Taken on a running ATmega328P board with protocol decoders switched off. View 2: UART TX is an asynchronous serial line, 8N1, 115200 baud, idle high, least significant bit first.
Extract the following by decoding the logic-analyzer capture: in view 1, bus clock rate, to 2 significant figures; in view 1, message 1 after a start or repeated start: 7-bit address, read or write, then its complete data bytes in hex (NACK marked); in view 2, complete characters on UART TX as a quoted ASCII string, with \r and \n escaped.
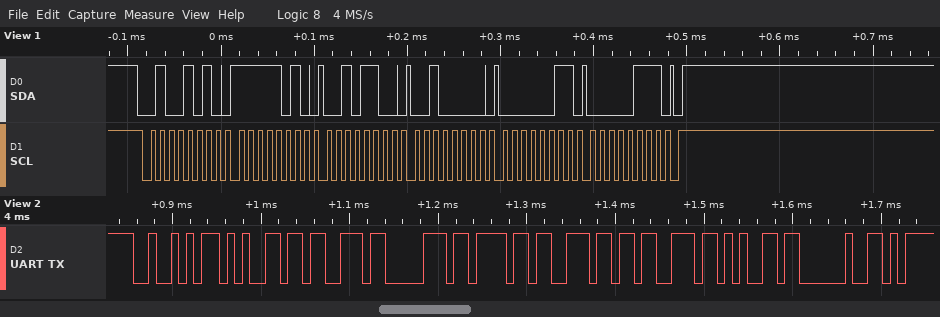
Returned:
100 kHz
0x25 write: FA 2C 20 03 07
"Response "
